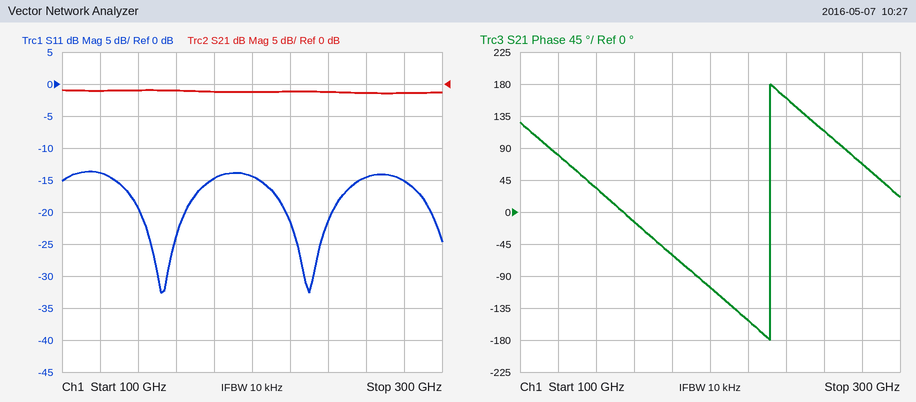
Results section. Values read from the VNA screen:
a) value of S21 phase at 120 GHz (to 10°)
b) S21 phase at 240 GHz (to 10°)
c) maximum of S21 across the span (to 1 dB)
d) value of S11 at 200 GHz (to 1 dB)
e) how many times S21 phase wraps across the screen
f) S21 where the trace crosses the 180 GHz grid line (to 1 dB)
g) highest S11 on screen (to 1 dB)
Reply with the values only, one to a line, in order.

80°
160°
-1 dB
-14 dB
1
-1 dB
-14 dB
